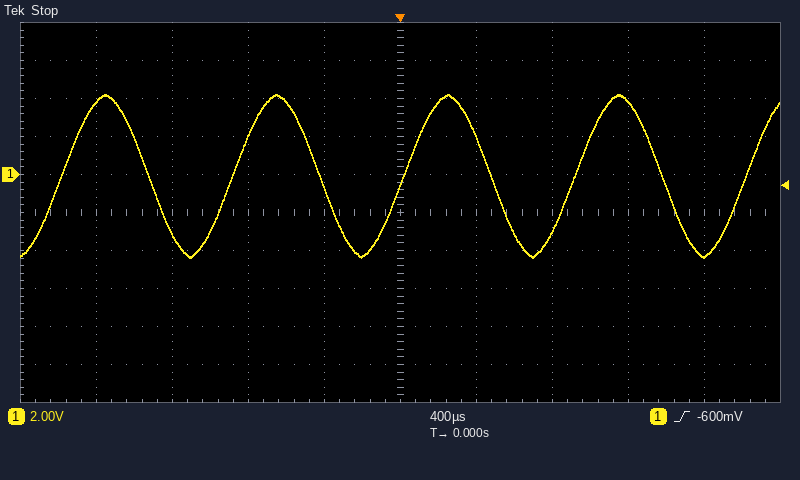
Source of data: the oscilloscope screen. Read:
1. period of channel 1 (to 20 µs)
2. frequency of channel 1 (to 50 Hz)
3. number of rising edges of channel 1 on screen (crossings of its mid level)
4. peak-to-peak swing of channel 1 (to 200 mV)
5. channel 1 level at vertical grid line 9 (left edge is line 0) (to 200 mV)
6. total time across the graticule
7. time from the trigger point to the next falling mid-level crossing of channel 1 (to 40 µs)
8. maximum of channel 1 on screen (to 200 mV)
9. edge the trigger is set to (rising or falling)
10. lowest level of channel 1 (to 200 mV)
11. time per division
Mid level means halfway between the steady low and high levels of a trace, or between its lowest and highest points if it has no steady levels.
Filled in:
900 µs
1.10 kHz
5
8.6 V
-4.2 V
4 ms
480 µs
4.2 V
rising
-4.4 V
400 µs
